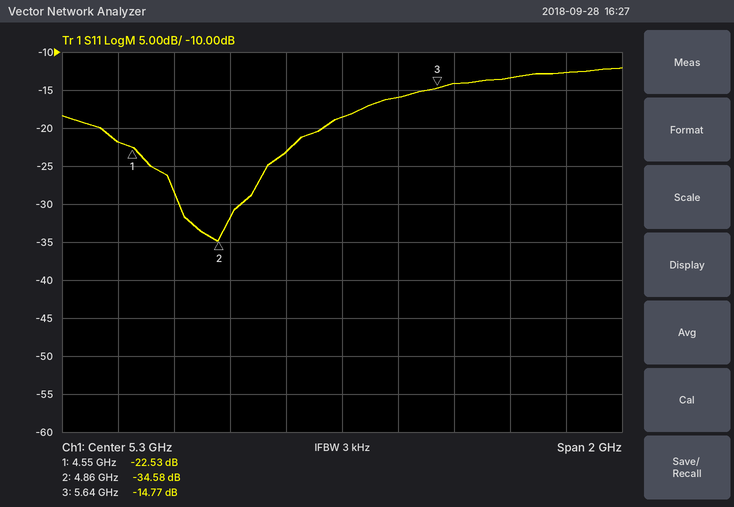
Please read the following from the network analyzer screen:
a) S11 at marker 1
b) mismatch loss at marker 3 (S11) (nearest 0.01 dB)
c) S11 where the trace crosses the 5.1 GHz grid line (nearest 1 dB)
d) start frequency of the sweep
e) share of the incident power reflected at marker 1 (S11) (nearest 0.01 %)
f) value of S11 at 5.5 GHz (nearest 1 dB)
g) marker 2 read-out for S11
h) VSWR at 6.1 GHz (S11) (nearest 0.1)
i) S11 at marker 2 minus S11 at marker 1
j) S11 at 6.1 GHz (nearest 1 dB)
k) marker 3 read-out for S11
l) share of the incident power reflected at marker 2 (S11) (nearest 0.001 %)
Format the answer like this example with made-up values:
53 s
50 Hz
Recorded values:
-22.53 dB
0.15 dB
-23 dB
4.3 GHz
0.56 %
-16 dB
-34.58 dB
1.6
-12.05 dB
-13 dB
-14.77 dB
0.035 %
